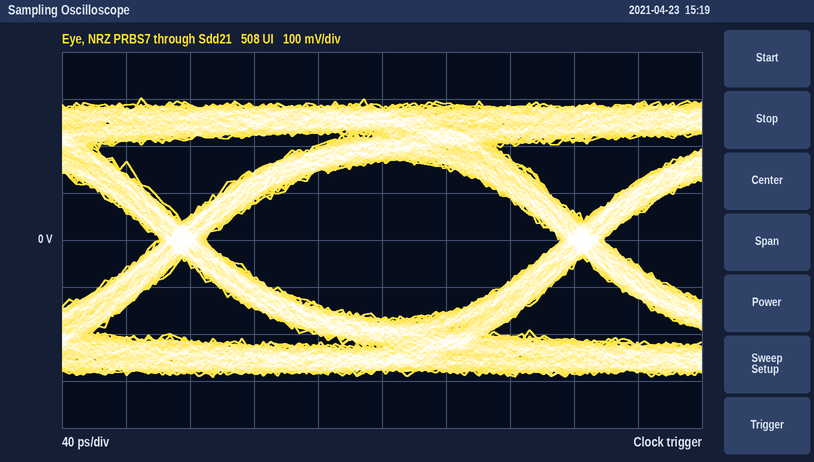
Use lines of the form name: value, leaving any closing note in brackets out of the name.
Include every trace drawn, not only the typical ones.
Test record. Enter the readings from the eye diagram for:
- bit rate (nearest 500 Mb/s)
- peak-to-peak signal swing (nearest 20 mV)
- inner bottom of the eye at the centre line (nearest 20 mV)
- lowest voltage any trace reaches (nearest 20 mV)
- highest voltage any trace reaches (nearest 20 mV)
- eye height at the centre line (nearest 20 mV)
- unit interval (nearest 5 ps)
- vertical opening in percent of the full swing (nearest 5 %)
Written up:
bit rate: 4.0 Gb/s
peak-to-peak signal swing: 600 mV
inner bottom of the eye at the centre line: -160 mV
lowest voltage any trace reaches: -300 mV
highest voltage any trace reaches: 300 mV
eye height at the centre line: 340 mV
unit interval: 250 ps
vertical opening in percent of the full swing: 55 %
